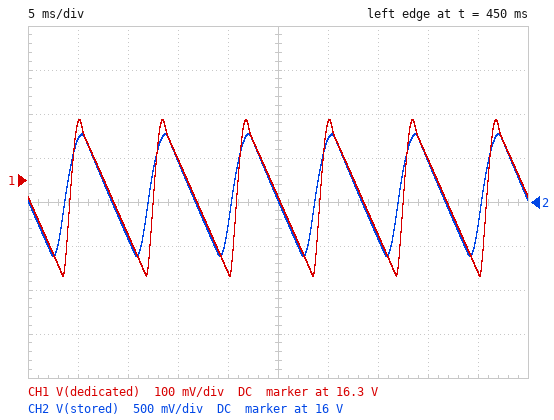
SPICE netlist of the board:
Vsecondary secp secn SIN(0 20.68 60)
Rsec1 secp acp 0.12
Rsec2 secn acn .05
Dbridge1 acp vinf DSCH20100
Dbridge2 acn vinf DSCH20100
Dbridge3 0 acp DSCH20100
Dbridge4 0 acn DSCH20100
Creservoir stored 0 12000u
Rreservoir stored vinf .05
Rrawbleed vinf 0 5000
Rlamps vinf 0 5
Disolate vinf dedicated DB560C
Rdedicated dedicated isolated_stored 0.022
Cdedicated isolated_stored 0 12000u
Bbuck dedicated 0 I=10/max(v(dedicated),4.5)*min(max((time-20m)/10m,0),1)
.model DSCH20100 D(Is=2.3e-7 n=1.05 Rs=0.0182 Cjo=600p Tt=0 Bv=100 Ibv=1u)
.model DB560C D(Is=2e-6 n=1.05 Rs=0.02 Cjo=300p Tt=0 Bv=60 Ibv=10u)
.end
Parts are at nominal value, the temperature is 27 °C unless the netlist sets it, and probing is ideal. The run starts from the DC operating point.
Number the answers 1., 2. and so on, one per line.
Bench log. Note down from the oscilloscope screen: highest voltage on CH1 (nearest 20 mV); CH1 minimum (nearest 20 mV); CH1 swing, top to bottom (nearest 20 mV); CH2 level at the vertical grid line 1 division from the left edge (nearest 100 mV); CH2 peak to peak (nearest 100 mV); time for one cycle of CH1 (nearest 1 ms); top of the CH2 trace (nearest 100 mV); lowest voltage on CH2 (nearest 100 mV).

1. 16.44 V
2. 16.08 V
3. 360 mV
4. 16.7 V
5. 1.4 V
6. 8 ms
7. 16.8 V
8. 15.4 V
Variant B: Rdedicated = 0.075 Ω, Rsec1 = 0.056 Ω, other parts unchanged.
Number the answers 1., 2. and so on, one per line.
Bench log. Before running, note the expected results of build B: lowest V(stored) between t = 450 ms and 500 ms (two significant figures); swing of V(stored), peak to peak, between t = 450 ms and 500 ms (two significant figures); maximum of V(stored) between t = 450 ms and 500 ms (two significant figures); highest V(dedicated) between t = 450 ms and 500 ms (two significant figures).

1. 16 V
2. 1.5 V
3. 17 V
4. 17 V
